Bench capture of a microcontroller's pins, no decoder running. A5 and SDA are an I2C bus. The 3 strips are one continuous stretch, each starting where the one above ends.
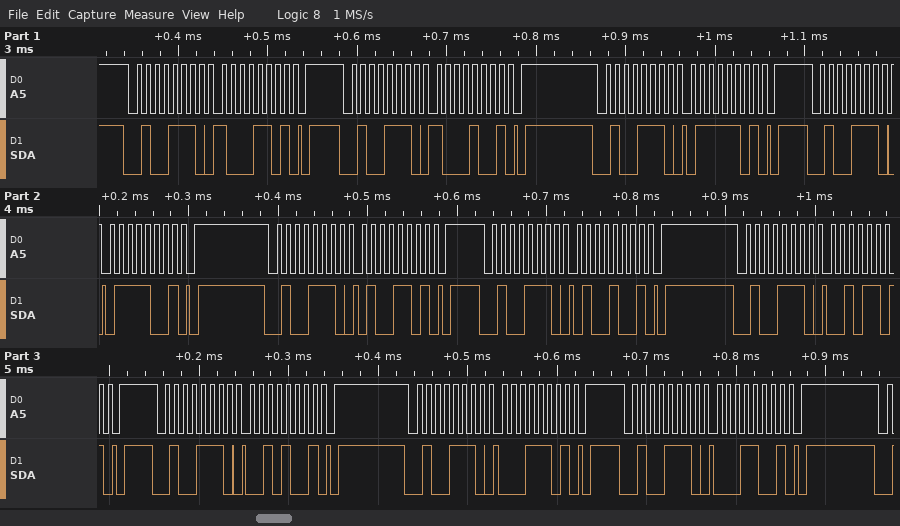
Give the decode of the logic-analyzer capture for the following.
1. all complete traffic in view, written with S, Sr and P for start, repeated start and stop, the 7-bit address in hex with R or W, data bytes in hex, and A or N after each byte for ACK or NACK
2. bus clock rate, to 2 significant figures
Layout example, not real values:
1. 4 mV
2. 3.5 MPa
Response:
1. S 27W A 8D A P S 27W A 89 A P S 27W A 7D A P S 27W A 79 A P S 27W A 4D A P S 27W A 49 A P S 27W A 2D A P S 27W A 29 A P S 27W A 1D A P S 27W A 19 A P
2. 100 kHz
